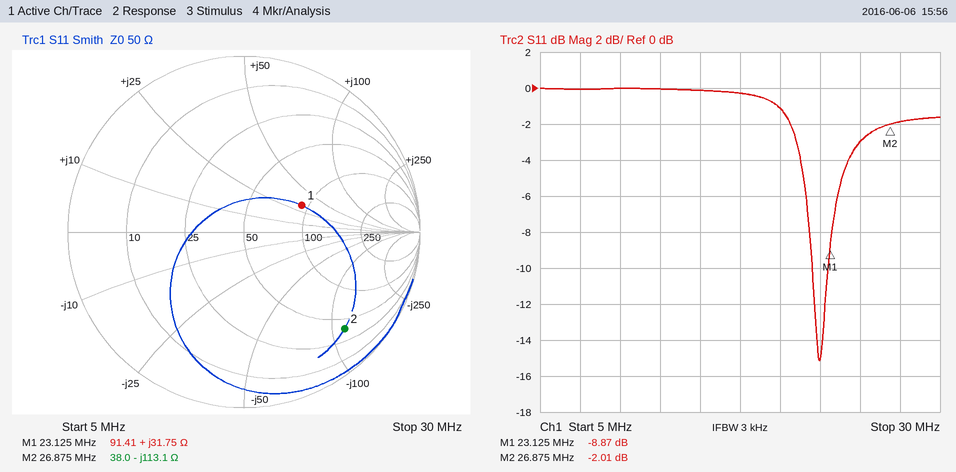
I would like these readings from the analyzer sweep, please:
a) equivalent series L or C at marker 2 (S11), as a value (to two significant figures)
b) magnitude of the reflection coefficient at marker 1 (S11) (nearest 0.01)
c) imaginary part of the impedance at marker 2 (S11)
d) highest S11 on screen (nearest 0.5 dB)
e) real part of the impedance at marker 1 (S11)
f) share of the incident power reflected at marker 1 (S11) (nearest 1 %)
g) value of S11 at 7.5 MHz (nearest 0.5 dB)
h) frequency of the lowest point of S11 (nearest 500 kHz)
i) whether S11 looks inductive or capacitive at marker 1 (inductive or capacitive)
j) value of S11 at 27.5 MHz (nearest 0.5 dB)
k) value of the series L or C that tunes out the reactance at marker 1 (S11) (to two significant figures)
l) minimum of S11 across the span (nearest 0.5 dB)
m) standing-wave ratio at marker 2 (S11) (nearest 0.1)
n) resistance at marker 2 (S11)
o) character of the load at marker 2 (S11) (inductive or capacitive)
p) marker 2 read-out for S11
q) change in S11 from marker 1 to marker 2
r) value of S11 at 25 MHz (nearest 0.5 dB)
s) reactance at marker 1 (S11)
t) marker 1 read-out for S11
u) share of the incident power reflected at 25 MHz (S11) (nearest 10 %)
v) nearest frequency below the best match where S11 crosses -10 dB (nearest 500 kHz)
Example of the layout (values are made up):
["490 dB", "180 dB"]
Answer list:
["52 pF", "0.36", "-113.1 Ω", "0.0 dB", "91.41 Ω", "13 %", "0.0 dB", "22.5 MHz", "inductive", "-2.0 dB", "220 pF", "-15.0 dB", "8.7", "38.0 Ω", "capacitive", "-2.01 dB", "6.86 dB", "-3.0 dB", "+31.75 Ω", "-8.87 dB", "50 %", "22.0 MHz"]
